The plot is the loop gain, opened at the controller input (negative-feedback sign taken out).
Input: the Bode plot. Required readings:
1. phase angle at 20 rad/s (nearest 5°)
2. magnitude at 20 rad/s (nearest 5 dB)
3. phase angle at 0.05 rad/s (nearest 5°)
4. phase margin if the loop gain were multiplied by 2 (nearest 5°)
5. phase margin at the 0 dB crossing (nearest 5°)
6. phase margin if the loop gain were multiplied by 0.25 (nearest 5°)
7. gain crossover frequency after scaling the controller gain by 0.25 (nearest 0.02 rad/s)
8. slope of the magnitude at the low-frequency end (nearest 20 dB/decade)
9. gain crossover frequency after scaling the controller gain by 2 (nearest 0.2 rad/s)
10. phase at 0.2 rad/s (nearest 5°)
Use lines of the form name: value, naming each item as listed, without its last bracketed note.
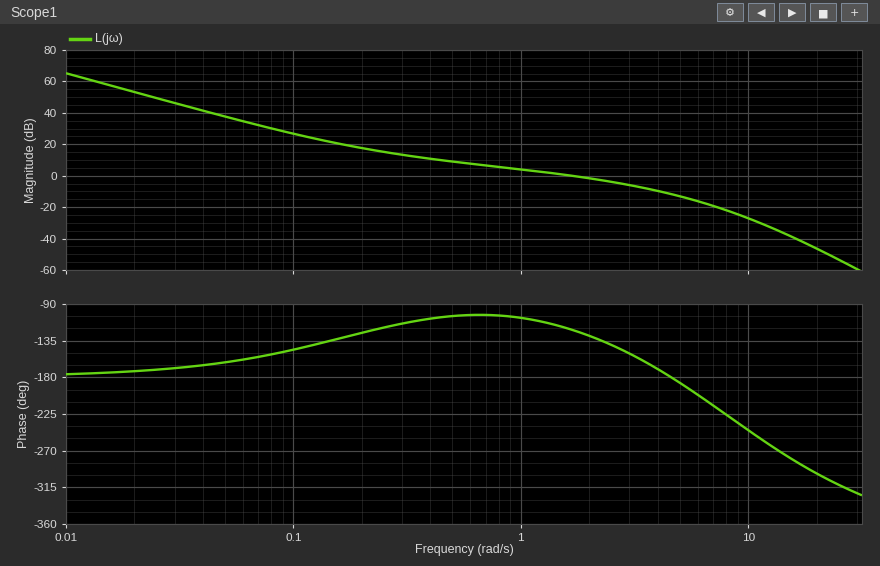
phase angle at 20 rad/s: -300°
magnitude at 20 rad/s: -45 dB
phase angle at 0.05 rad/s: -160°
phase margin if the loop gain were multiplied by 2: 30°
phase margin at the 0 dB crossing: 60°
phase margin if the loop gain were multiplied by 0.25: 70°
gain crossover frequency after scaling the controller gain by 0.25: 0.34 rad/s
slope of the magnitude at the low-frequency end: -40 dB/decade
gain crossover frequency after scaling the controller gain by 2: 3.0 rad/s
phase at 0.2 rad/s: -125°
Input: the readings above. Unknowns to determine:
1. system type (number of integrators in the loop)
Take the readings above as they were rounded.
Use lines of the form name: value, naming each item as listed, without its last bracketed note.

system type: 2
